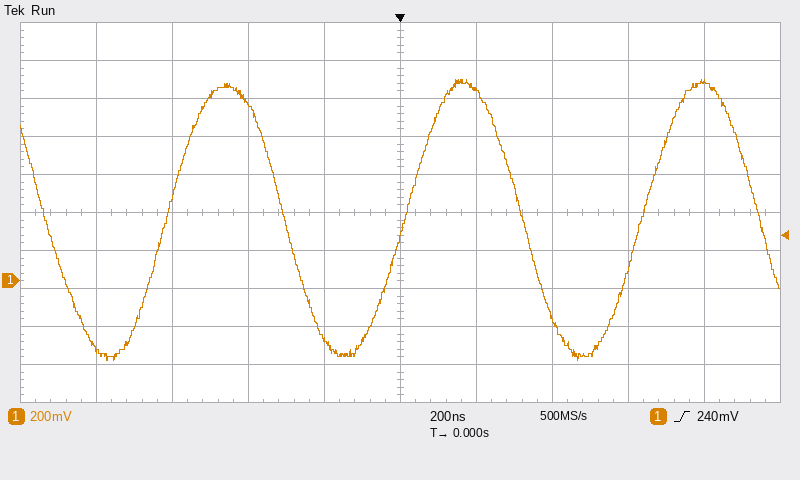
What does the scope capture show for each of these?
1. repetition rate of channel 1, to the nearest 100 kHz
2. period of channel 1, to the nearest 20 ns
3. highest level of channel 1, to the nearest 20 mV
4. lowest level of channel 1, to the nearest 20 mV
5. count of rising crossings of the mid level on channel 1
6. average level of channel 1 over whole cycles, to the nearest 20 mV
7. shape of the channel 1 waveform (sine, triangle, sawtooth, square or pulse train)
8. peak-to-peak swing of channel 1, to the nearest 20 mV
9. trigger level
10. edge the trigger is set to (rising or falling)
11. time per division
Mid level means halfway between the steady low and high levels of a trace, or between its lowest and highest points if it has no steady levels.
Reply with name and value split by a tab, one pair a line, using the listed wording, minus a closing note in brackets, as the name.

repetition rate of channel 1, to the nearest 100 kHz	1.6 MHz
period of channel 1, to the nearest 20 ns	620 ns
highest level of channel 1, to the nearest 20 mV	1.06 V
lowest level of channel 1, to the nearest 20 mV	-420 mV
count of rising crossings of the mid level on channel 1	3
average level of channel 1 over whole cycles, to the nearest 20 mV	320 mV
shape of the channel 1 waveform	sine
peak-to-peak swing of channel 1, to the nearest 20 mV	1.48 V
trigger level	240 mV
edge the trigger is set to	rising
time per division	200 ns
